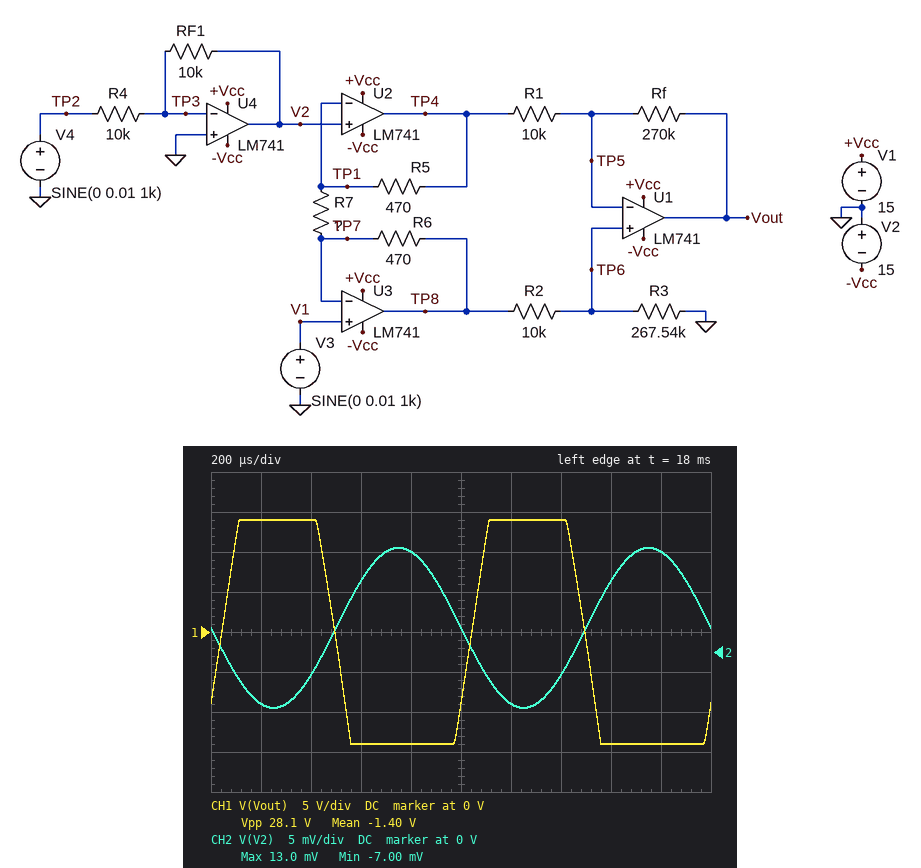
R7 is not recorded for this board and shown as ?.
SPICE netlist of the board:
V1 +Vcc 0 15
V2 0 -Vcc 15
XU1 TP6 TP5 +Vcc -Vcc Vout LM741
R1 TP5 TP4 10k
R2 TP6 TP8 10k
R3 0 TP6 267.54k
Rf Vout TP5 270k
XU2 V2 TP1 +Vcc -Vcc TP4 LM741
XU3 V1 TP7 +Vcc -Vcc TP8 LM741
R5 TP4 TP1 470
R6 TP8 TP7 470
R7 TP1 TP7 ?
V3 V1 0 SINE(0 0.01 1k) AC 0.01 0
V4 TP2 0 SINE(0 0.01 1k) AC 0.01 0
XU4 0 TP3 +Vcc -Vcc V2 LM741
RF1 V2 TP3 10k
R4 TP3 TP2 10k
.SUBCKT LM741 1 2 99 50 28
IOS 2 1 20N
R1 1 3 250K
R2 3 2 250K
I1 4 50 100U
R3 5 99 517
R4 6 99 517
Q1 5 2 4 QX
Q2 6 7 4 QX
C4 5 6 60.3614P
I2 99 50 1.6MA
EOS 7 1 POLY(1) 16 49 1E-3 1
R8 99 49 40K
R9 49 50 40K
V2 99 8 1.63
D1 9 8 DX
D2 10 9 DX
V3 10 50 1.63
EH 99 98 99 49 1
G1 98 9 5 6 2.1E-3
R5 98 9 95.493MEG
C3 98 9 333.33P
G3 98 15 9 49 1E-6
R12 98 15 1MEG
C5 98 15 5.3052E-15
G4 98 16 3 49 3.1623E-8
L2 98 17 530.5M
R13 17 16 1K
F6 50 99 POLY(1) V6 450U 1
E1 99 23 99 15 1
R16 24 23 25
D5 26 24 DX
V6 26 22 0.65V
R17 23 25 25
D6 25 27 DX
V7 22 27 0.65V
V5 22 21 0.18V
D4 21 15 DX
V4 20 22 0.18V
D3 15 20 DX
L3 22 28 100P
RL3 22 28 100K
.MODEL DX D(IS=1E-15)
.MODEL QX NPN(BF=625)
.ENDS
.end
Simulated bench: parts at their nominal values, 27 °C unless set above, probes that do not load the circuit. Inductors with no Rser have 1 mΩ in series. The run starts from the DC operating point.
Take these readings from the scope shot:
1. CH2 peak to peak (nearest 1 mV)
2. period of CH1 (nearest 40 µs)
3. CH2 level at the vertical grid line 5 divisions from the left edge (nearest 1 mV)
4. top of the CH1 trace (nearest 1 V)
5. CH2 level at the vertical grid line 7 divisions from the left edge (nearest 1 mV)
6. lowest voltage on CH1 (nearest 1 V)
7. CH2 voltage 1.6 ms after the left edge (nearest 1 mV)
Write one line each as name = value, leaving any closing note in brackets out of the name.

CH2 peak to peak = 20 mV
period of CH1 = 1.00 ms
CH2 level at the vertical grid line 5 divisions from the left edge = 3 mV
top of the CH1 trace = 14 V
CH2 level at the vertical grid line 7 divisions from the left edge = -3 mV
lowest voltage on CH1 = -14 V
CH2 voltage 1.6 ms after the left edge = 9 mV
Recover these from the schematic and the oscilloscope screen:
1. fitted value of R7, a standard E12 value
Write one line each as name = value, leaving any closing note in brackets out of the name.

fitted value of R7, a standard E12 value = 15 Ω
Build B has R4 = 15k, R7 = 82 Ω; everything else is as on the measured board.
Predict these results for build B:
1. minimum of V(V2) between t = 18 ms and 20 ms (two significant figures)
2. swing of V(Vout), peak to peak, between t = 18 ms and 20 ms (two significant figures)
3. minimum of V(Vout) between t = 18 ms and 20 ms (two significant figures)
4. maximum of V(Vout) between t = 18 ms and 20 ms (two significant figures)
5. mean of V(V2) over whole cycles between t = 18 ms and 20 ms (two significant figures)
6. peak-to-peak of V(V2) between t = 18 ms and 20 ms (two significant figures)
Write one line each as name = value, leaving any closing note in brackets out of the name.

minimum of V(V2) between t = 18 ms and 20 ms = -4.0 mV
swing of V(Vout), peak to peak, between t = 18 ms and 20 ms = 11 V
minimum of V(Vout) between t = 18 ms and 20 ms = -6.5 V
maximum of V(Vout) between t = 18 ms and 20 ms = 4.7 V
mean of V(V2) over whole cycles between t = 18 ms and 20 ms = 2.7 mV
peak-to-peak of V(V2) between t = 18 ms and 20 ms = 13 mV
